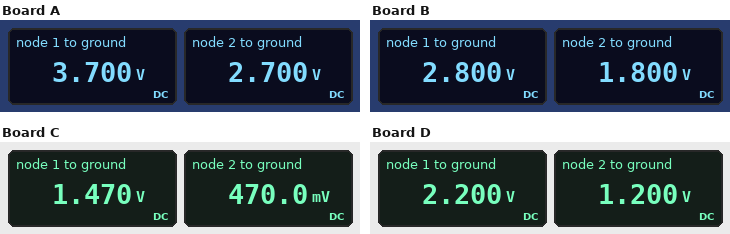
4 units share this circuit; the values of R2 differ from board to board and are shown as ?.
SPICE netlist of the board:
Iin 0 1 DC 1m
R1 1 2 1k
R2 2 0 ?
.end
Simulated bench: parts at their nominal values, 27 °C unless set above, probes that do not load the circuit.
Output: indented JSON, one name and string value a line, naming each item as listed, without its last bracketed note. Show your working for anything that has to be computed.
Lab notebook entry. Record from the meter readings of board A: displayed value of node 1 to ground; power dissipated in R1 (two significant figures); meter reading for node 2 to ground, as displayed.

{
  "displayed value of node 1 to ground": "3.700 V",
  "power dissipated in R1": "(3.7 V - 2.7 V)^2 / 1 kΩ = 1.0 mW",
  "meter reading for node 2 to ground, as displayed": "2.700 V"
}
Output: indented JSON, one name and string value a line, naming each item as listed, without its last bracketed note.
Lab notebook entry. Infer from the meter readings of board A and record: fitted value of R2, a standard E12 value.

{
  "fitted value of R2, a standard E12 value": "2.7 kΩ"
}
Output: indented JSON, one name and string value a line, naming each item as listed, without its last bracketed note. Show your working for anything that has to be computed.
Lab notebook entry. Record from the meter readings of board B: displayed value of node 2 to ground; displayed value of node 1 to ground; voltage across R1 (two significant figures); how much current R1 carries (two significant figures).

{
  "displayed value of node 2 to ground": "1.800 V",
  "displayed value of node 1 to ground": "2.800 V",
  "voltage across R1": "2.8 V - 1.8 V = 1.0 V",
  "how much current R1 carries": "(2.8 V - 1.8 V) / 1 kΩ = 1.0 mA"
}
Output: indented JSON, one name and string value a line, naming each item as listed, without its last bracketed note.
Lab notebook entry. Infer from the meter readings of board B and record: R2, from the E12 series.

{
  "R2, from the E12 series": "1.8 kΩ"
}
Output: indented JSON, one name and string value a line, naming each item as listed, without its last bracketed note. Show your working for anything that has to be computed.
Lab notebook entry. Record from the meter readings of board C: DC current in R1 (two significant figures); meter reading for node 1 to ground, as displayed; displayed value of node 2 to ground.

{
  "DC current in R1": "(1.47 V - 470 mV) / 1 kΩ = 1.0 mA",
  "meter reading for node 1 to ground, as displayed": "1.470 V",
  "displayed value of node 2 to ground": "470.0 mV"
}
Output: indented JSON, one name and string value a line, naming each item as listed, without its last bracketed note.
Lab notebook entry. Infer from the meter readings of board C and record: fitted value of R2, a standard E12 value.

{
  "fitted value of R2, a standard E12 value": "470 Ω"
}
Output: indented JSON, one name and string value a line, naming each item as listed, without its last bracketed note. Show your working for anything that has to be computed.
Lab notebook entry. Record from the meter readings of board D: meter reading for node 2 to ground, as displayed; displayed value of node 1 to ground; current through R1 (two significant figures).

{
  "meter reading for node 2 to ground, as displayed": "1.200 V",
  "displayed value of node 1 to ground": "2.200 V",
  "current through R1": "(2.2 V - 1.2 V) / 1 kΩ = 1.0 mA"
}
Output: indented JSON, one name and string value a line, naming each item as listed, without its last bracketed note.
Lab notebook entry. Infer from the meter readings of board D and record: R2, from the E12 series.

{
  "R2, from the E12 series": "1.2 kΩ"
}
